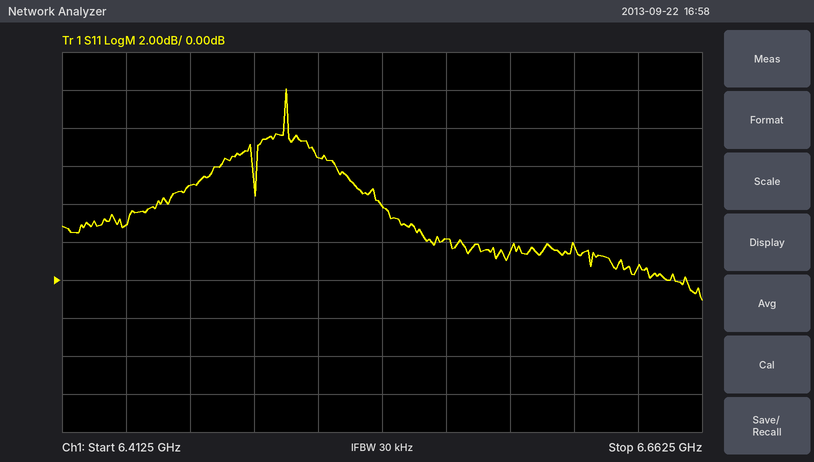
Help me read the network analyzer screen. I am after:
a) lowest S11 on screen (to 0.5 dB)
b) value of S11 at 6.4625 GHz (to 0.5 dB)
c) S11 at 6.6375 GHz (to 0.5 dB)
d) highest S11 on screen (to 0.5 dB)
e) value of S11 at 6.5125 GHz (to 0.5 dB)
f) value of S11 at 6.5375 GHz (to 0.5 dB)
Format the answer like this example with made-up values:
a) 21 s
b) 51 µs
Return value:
a) -1.0 dB
b) 5.0 dB
c) 0.5 dB
d) 10.0 dB
e) 6.5 dB
f) 4.0 dB
